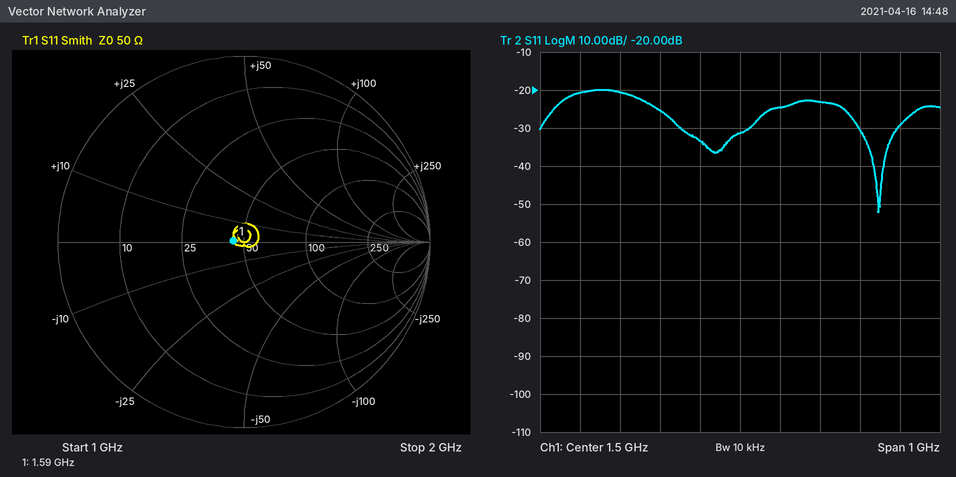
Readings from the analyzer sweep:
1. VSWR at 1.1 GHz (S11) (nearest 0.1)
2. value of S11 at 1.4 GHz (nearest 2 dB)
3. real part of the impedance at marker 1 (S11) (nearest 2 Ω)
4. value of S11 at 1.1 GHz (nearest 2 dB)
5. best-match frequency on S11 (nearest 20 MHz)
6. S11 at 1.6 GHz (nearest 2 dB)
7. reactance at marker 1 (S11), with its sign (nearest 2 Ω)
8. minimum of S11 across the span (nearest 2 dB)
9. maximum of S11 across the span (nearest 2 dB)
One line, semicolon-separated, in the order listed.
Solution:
1.2; -34 dB; 44 Ω; -20 dB; 1.84 GHz; -24 dB; 0 Ω; -52 dB; -20 dB
